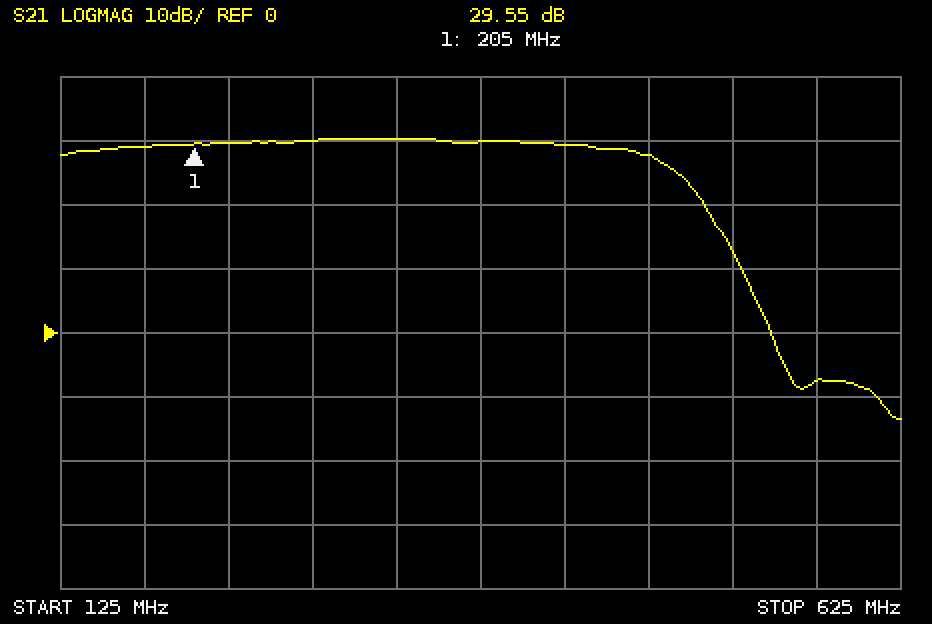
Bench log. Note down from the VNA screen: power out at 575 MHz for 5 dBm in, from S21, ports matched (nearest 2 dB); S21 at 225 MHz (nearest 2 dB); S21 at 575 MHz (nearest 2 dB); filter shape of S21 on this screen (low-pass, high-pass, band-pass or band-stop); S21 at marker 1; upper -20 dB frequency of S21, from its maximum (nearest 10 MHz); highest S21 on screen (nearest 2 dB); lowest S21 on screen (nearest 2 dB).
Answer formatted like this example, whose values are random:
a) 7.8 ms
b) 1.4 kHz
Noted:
a) -2 dBm
b) 30 dB
c) -8 dB
d) low-pass
e) 29.55 dB
f) 530 MHz
g) 30 dB
h) -14 dB
